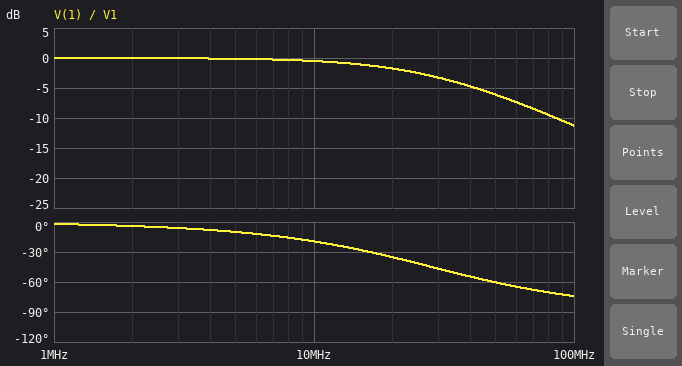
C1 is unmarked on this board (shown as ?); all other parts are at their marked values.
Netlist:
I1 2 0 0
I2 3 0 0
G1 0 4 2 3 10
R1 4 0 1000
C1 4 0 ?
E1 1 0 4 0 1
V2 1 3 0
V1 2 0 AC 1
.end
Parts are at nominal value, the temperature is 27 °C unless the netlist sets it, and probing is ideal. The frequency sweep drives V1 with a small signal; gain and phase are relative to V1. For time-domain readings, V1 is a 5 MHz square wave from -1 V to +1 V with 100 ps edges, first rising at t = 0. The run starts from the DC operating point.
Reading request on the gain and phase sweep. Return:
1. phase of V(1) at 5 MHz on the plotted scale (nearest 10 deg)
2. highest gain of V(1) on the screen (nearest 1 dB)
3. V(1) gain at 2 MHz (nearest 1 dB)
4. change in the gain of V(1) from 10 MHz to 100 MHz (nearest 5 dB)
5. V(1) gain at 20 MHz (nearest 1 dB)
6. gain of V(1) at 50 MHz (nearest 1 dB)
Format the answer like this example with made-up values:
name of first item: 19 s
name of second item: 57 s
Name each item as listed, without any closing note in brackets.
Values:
phase of V(1) at 5 MHz on the plotted scale: -10 deg
highest gain of V(1) on the screen: 0 dB
V(1) gain at 2 MHz: 0 dB
change in the gain of V(1) from 10 MHz to 100 MHz: -10 dB
V(1) gain at 20 MHz: -2 dB
gain of V(1) at 50 MHz: -6 dB
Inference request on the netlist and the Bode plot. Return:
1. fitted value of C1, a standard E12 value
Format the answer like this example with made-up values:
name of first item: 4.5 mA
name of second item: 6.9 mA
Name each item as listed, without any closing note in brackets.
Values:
fitted value of C1, a standard E12 value: 56 nF
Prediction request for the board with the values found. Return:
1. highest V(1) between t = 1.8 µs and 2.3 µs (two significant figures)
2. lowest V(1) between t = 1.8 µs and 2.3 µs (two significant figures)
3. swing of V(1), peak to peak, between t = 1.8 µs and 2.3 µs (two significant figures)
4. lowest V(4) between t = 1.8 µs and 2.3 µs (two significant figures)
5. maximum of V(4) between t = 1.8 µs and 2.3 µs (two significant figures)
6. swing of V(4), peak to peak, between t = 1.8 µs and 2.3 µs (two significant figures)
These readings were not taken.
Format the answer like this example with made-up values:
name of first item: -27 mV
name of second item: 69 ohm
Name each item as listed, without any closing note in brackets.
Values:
highest V(1) between t = 1.8 µs and 2.3 µs: 1.0 V
lowest V(1) between t = 1.8 µs and 2.3 µs: -1.0 V
swing of V(1), peak to peak, between t = 1.8 µs and 2.3 µs: 2.0 V
lowest V(4) between t = 1.8 µs and 2.3 µs: -1.0 V
maximum of V(4) between t = 1.8 µs and 2.3 µs: 1.0 V
swing of V(4), peak to peak, between t = 1.8 µs and 2.3 µs: 2.0 V
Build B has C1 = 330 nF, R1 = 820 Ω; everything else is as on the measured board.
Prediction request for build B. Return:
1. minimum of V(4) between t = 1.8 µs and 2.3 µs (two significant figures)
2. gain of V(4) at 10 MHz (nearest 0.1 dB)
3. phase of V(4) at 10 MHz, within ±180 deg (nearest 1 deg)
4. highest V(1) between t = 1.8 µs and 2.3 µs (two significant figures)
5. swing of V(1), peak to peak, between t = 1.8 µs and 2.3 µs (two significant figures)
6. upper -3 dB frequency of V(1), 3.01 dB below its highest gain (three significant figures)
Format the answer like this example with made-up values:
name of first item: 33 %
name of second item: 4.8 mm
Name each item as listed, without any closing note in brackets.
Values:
minimum of V(4) between t = 1.8 µs and 2.3 µs: -910 mV
gain of V(4) at 10 MHz: -7.2 dB
phase of V(4) at 10 MHz, within ±180 deg: -64 deg
highest V(1) between t = 1.8 µs and 2.3 µs: 910 mV
swing of V(1), peak to peak, between t = 1.8 µs and 2.3 µs: 1.8 V
upper -3 dB frequency of V(1), 3.01 dB below its highest gain: 4.82 MHz
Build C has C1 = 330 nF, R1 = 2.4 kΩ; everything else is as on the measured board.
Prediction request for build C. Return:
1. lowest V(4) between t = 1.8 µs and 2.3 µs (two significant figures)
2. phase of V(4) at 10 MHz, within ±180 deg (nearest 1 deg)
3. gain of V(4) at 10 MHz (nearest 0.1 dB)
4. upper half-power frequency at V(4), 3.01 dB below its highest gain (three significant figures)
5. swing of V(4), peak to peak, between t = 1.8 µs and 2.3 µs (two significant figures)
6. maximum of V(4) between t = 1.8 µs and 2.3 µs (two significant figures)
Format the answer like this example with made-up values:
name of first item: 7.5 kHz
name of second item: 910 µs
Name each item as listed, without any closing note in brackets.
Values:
lowest V(4) between t = 1.8 µs and 2.3 µs: -910 mV
phase of V(4) at 10 MHz, within ±180 deg: -64 deg
gain of V(4) at 10 MHz: -7.2 dB
upper half-power frequency at V(4), 3.01 dB below its highest gain: 4.82 MHz
swing of V(4), peak to peak, between t = 1.8 µs and 2.3 µs: 1.8 V
maximum of V(4) between t = 1.8 µs and 2.3 µs: 910 mV
